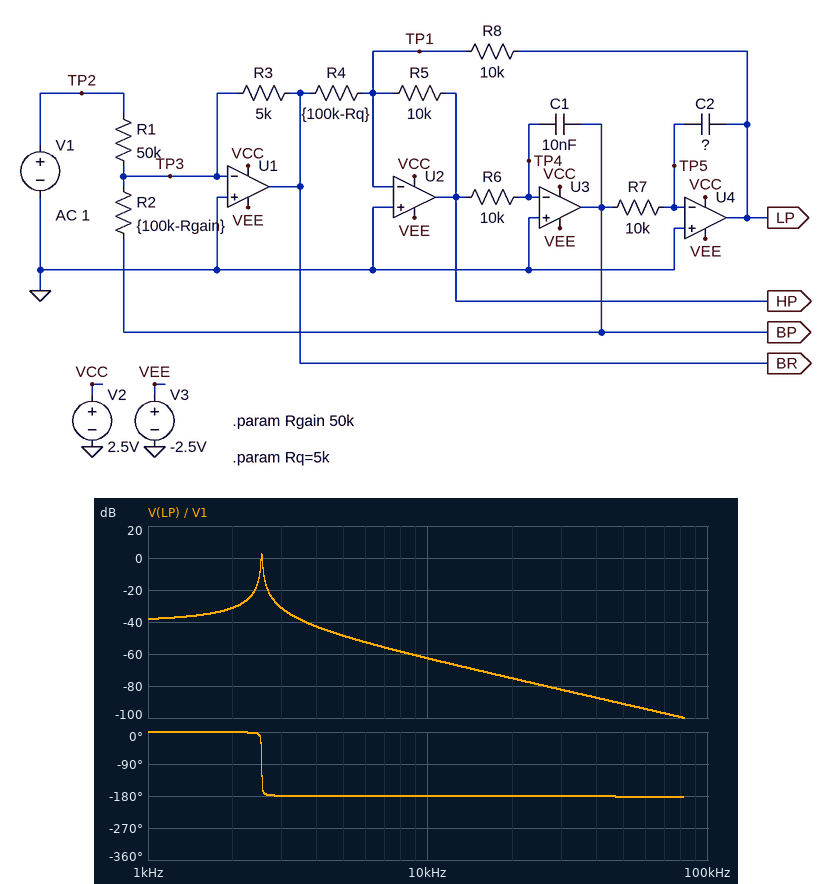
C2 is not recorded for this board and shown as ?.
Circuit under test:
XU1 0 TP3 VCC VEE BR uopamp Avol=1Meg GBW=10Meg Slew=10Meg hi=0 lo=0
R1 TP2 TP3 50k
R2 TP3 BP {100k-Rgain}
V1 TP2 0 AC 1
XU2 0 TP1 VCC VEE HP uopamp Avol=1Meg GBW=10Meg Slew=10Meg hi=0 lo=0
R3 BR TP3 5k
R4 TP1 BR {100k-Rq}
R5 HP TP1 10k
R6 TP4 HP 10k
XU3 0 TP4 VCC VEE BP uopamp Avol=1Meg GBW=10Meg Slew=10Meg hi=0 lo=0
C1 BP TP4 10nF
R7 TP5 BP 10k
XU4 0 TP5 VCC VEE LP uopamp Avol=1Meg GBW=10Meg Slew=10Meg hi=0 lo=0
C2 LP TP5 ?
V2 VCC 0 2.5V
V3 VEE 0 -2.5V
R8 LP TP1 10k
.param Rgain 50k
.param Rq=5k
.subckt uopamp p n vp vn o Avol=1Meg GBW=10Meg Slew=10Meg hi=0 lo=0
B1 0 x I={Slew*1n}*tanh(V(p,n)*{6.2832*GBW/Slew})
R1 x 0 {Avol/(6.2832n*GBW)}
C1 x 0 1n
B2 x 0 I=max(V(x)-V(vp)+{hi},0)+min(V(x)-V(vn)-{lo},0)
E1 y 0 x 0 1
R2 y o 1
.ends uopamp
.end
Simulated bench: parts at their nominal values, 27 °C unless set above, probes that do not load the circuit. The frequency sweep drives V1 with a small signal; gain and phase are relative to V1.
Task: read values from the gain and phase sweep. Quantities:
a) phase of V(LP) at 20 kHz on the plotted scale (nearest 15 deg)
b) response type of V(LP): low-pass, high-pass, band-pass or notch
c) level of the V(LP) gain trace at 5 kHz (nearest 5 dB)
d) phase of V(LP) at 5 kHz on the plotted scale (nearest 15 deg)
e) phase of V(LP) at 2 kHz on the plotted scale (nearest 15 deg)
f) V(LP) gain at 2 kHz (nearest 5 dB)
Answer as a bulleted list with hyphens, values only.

- -180 deg
- band-pass
- -50 dB
- -180 deg
- 0 deg
- -30 dB
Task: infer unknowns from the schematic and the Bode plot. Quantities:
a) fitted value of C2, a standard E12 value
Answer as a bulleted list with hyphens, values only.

- 3.9 nF
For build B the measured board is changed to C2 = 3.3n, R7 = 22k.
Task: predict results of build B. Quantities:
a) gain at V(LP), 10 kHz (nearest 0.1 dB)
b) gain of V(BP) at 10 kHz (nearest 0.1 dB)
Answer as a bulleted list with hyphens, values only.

- -68.4 dB
- -55.2 dB
